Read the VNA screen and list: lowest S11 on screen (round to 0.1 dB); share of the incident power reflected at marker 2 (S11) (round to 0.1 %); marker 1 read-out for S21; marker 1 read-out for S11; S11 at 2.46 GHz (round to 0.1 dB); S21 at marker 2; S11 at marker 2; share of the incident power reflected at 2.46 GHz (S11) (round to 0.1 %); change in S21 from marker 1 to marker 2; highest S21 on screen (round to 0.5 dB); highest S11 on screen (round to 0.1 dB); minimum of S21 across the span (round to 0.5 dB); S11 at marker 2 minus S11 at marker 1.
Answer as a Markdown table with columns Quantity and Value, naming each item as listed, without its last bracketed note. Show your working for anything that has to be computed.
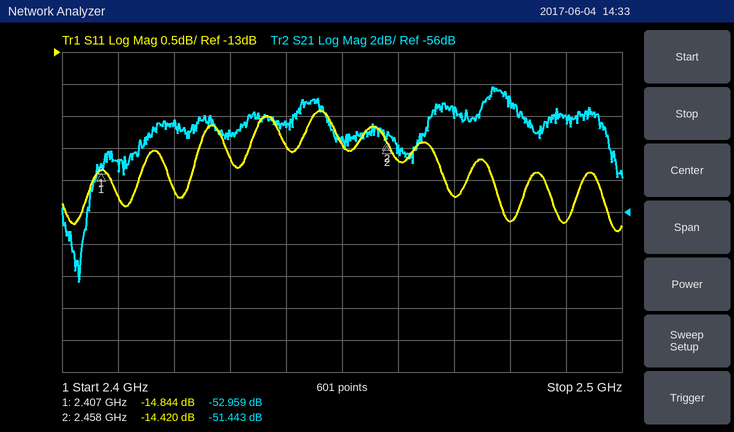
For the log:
| Quantity | Value |
|---|---|
| lowest S11 on screen | -15.8 dB |
| share of the incident power reflected at marker 2 (S11) | 10^(-14.42/10) ≈ 3.6 % |
| marker 1 read-out for S21 | -52.959 dB |
| marker 1 read-out for S11 | -14.844 dB |
| S11 at 2.46 GHz | -14.7 dB |
| S21 at marker 2 | -51.443 dB |
| S11 at marker 2 | -14.420 dB |
| share of the incident power reflected at 2.46 GHz (S11) | 10^(-14.7/10) ≈ 3.4 % |
| change in S21 from marker 1 to marker 2 | -51.443 − (-52.959) = 1.516 dB |
| highest S21 on screen | -48.0 dB |
| highest S11 on screen | -13.9 dB |
| minimum of S21 across the span | -60.5 dB |
| S11 at marker 2 minus S11 at marker 1 | -14.42 − (-14.844) = 0.424 dB |
